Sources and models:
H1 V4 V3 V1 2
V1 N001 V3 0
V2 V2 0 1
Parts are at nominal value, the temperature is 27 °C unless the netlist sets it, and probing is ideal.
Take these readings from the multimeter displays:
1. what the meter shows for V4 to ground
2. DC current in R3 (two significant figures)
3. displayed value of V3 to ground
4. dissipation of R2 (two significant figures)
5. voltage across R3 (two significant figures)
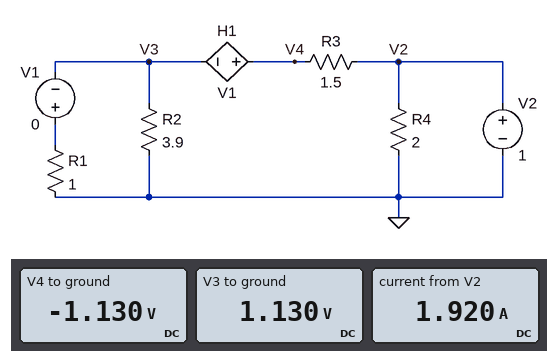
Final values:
-1.130 V
1.4 A
1.130 V
330 mW
2.1 V
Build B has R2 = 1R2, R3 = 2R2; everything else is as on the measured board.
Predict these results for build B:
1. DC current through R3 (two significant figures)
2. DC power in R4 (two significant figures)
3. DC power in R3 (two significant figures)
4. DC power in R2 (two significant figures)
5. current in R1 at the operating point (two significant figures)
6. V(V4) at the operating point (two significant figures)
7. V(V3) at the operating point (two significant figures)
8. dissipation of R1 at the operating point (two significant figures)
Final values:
600 mA
500 mW
800 mW
91 mW
330 mA
-330 mV
330 mV
110 mW
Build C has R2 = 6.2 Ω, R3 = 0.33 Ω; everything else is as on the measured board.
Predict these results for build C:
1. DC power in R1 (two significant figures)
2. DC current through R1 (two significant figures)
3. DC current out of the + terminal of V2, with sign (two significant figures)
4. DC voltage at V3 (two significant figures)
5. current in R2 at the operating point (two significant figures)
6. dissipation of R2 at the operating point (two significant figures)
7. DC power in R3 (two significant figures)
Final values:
2.6 W
1.6 A
-1.4 A
-1.6 V
260 mA
420 mW
1.2 W
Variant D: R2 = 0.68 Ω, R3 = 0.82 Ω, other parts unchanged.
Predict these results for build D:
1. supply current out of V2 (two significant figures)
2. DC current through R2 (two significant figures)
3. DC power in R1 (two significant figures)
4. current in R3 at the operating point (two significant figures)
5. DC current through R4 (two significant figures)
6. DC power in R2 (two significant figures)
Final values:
2.9 A
1.4 A
950 mW
2.4 A
500 mA
1.4 W
